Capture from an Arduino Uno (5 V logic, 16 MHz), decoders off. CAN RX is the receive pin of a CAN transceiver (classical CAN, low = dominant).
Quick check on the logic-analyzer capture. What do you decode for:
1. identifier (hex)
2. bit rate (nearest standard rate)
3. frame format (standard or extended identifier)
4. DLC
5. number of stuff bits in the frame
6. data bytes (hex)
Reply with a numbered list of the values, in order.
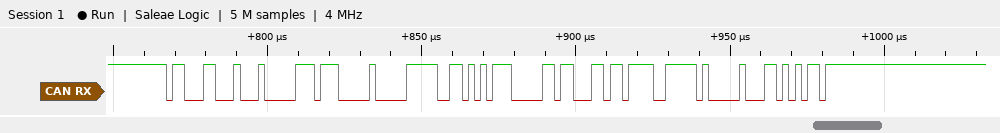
1. 0x631
2. 500 kbit/s
3. standard
4. 8
5. 7
6. 37 00 3D AB 82 C6 DE 7E
